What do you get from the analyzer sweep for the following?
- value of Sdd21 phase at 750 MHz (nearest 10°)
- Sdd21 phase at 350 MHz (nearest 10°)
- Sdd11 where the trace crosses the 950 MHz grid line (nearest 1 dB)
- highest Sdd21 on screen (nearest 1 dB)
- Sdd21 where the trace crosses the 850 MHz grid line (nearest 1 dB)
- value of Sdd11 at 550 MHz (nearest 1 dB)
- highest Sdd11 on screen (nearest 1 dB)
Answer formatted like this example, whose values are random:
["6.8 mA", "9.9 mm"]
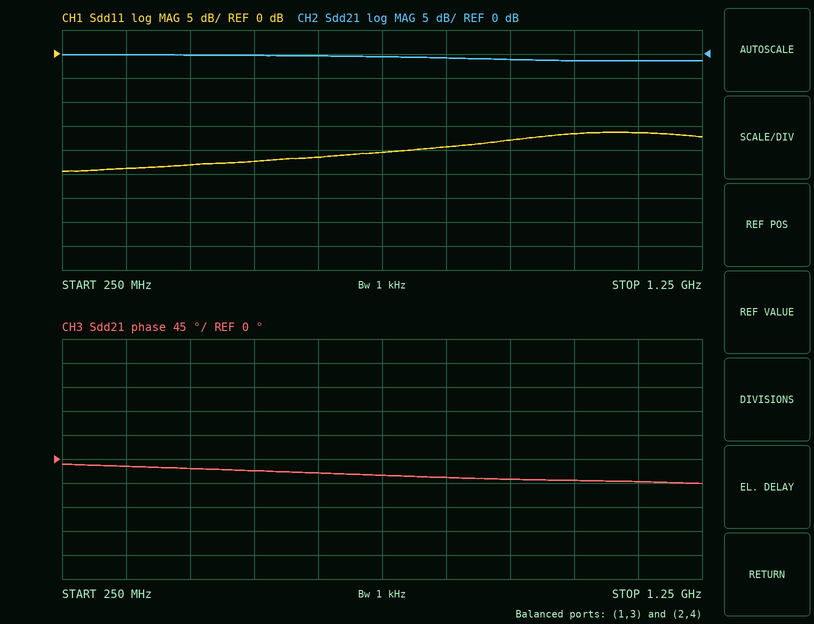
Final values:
["-30°", "-10°", "-18 dB", "0 dB", "-1 dB", "-22 dB", "-16 dB"]
